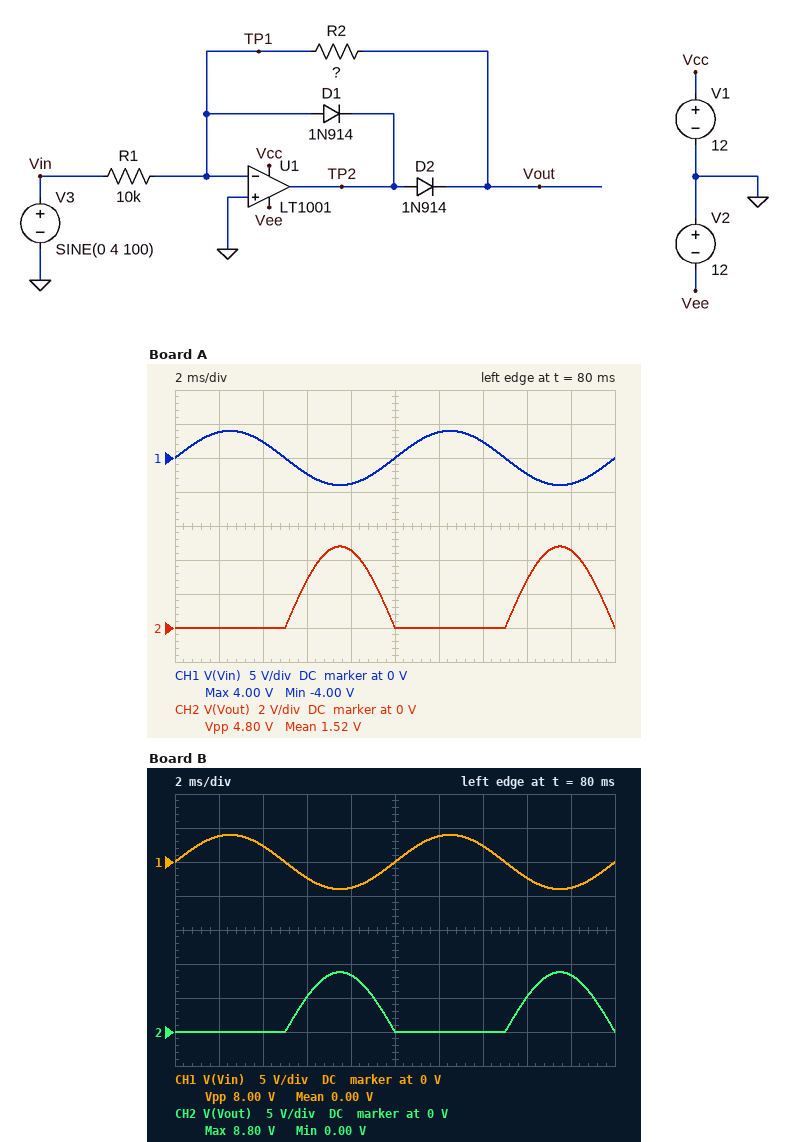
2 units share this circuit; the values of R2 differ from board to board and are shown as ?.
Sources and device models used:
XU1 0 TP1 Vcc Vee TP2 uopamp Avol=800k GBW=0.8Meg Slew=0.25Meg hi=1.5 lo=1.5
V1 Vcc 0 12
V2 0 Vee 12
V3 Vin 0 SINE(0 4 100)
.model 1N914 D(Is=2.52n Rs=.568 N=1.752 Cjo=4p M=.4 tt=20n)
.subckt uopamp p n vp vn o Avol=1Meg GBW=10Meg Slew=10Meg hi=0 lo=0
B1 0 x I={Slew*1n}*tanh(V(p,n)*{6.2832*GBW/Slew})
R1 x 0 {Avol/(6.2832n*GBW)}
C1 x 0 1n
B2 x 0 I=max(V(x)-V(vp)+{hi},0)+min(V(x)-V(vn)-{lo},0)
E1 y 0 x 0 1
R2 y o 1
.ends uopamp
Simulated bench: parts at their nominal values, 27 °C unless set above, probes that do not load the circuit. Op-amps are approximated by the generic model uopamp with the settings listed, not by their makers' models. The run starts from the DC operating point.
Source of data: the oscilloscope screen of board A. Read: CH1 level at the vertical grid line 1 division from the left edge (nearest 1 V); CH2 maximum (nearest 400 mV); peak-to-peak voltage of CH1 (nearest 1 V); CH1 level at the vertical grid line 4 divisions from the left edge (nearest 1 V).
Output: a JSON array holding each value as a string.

["4 V", "4.8 V", "8 V", "-4 V"]
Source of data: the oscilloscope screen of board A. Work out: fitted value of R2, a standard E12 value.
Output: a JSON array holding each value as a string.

["12 kΩ"]
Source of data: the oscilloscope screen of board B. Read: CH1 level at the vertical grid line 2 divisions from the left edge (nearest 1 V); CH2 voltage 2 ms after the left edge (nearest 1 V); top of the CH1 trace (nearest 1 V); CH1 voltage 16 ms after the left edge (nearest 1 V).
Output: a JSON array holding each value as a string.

["2 V", "0 V", "4 V", "-2 V"]
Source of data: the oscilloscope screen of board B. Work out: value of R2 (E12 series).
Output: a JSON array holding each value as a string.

["22 kΩ"]
